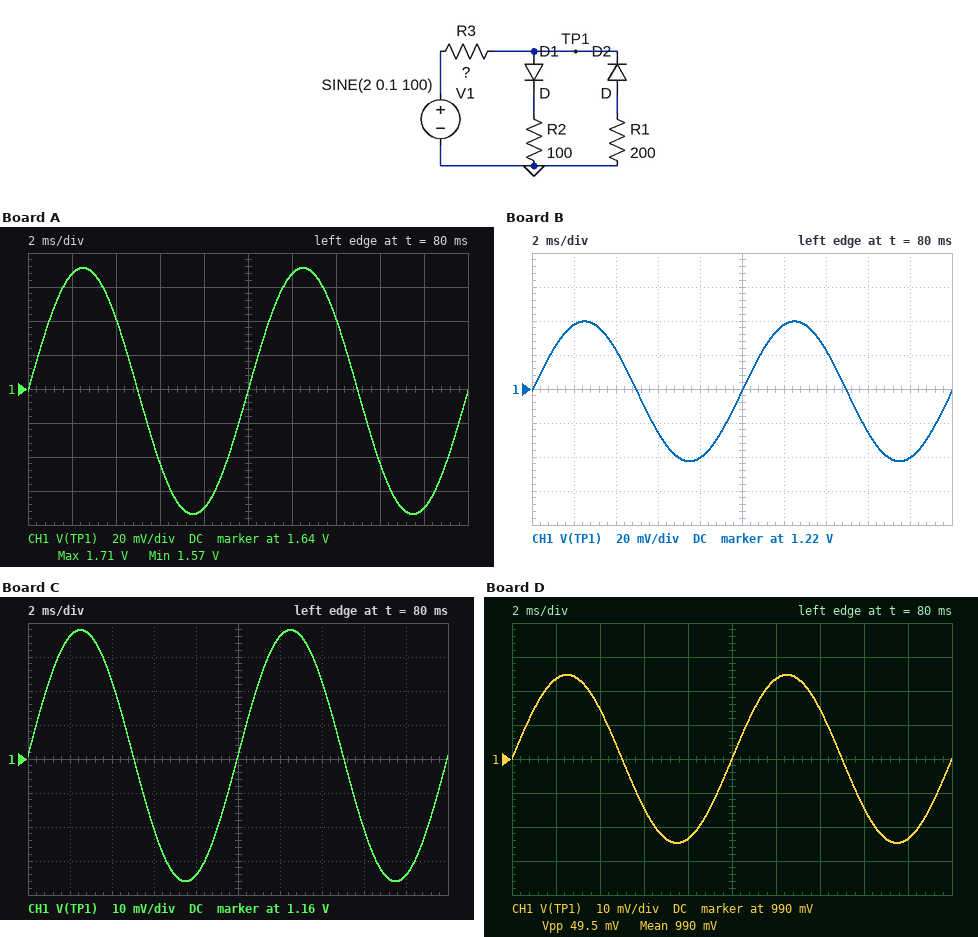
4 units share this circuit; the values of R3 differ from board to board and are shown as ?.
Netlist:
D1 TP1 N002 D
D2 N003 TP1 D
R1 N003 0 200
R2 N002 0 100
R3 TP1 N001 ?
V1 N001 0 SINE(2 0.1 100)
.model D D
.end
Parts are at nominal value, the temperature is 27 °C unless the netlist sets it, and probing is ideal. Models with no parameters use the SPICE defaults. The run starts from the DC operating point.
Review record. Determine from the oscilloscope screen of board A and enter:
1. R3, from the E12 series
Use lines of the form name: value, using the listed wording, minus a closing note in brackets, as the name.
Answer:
R3, from the E12 series: 39 Ω
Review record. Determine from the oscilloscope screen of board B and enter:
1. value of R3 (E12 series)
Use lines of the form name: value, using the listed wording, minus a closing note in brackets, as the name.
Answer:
value of R3: 150 Ω
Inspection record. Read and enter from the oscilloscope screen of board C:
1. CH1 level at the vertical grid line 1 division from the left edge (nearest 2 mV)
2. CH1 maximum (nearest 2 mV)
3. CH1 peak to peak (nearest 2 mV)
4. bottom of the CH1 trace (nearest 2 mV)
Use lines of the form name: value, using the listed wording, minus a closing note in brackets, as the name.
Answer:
CH1 level at the vertical grid line 1 division from the left edge: 1.196 V
CH1 maximum: 1.198 V
CH1 peak to peak: 74 mV
bottom of the CH1 trace: 1.124 V
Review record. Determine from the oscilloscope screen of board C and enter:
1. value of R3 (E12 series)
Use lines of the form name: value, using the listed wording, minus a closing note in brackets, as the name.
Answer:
value of R3: 180 Ω
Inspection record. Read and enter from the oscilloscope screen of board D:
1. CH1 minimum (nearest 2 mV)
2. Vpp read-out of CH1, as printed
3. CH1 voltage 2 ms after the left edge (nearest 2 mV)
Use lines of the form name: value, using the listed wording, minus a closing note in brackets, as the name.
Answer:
CH1 minimum: 966 mV
Vpp read-out of CH1, as printed: 49.5 mV
CH1 voltage 2 ms after the left edge: 1.014 V
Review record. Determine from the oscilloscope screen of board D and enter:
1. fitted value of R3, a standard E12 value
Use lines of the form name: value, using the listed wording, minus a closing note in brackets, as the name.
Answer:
fitted value of R3, a standard E12 value: 330 Ω
